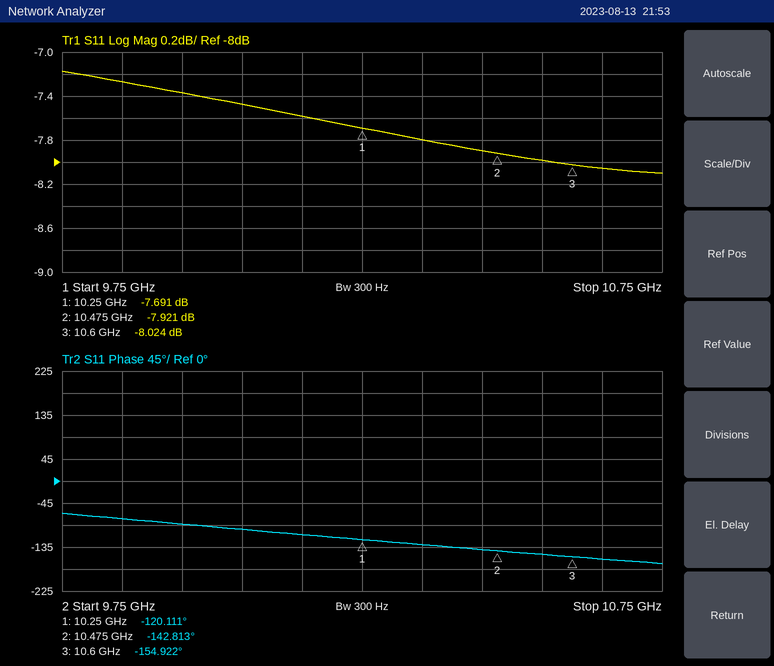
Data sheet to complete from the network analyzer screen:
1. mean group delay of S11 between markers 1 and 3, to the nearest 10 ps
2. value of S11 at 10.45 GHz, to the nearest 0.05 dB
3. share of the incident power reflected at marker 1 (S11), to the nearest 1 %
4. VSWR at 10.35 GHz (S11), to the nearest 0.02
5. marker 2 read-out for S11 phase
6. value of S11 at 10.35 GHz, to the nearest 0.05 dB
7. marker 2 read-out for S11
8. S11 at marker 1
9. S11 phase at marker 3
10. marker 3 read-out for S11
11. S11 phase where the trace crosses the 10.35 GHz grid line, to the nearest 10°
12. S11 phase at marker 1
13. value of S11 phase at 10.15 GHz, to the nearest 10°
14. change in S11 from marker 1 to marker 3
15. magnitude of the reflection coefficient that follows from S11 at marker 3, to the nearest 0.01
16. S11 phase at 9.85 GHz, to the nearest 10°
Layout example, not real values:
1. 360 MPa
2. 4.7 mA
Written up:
1. 280 ps
2. -7.90 dB
3. 17 %
4. 2.38
5. -142.813°
6. -7.80 dB
7. -7.921 dB
8. -7.691 dB
9. -154.922°
10. -8.024 dB
11. -130°
12. -120.111°
13. -110°
14. -0.333 dB
15. 0.40
16. -80°
